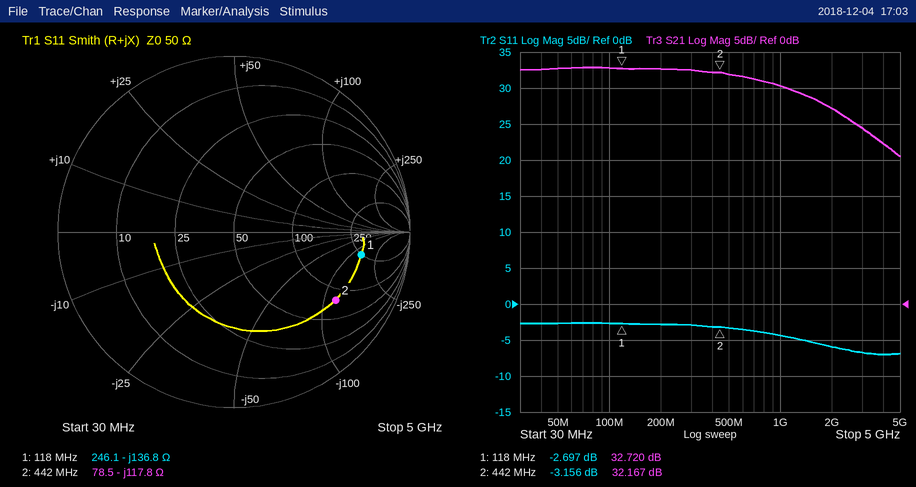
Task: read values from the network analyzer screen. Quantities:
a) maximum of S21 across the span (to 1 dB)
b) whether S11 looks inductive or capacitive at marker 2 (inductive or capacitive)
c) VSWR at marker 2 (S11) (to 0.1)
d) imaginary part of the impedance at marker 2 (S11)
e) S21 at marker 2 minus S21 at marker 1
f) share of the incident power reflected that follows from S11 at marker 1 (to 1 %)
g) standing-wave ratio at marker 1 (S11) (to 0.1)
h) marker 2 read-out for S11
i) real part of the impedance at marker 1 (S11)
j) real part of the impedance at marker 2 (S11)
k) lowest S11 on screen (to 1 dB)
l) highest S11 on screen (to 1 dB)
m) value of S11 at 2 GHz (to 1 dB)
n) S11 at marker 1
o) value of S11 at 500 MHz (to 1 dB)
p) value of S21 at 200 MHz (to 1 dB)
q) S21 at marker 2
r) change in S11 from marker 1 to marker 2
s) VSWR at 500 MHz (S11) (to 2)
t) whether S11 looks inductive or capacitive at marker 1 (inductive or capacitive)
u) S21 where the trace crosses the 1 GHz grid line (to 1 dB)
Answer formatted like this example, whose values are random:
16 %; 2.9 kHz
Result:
33 dB; capacitive; 5.6; -117.8 Ω; -0.553 dB; 54 %; 6.5; -3.156 dB; 246.1 Ω; 78.5 Ω; -7 dB; -3 dB; -6 dB; -2.697 dB; -3 dB; 33 dB; 32.167 dB; -0.459 dB; 6; capacitive; 30 dB
